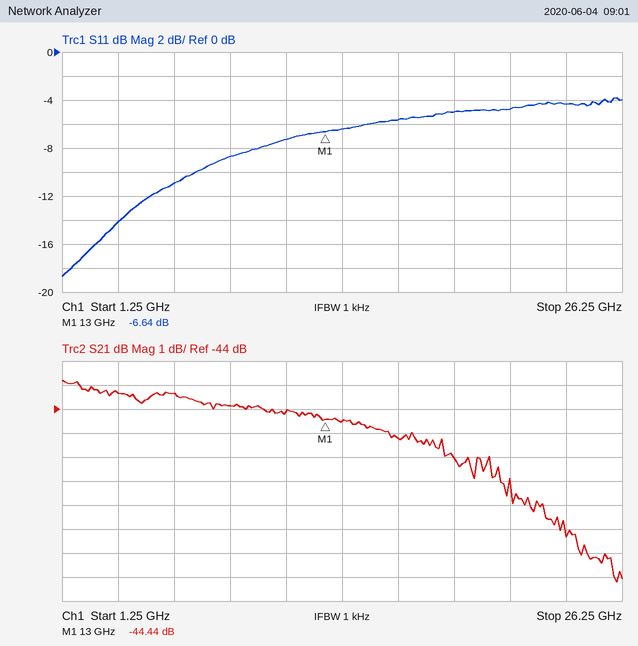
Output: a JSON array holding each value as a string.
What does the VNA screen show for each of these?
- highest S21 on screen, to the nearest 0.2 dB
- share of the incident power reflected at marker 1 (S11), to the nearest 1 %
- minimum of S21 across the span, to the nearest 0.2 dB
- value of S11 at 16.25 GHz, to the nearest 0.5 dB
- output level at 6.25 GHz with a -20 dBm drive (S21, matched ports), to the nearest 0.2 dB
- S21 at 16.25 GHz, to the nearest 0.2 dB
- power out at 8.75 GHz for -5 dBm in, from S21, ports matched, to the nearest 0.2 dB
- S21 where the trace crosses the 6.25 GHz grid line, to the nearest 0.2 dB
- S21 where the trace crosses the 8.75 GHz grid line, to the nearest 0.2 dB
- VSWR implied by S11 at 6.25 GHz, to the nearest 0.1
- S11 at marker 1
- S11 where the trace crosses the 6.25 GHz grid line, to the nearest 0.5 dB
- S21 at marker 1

["-42.8 dB", "22 %", "-51.2 dB", "-5.5 dB", "-63.4 dBm", "-45.2 dB", "-48.8 dBm", "-43.4 dB", "-43.8 dB", "1.8", "-6.64 dB", "-11.0 dB", "-44.44 dB"]
